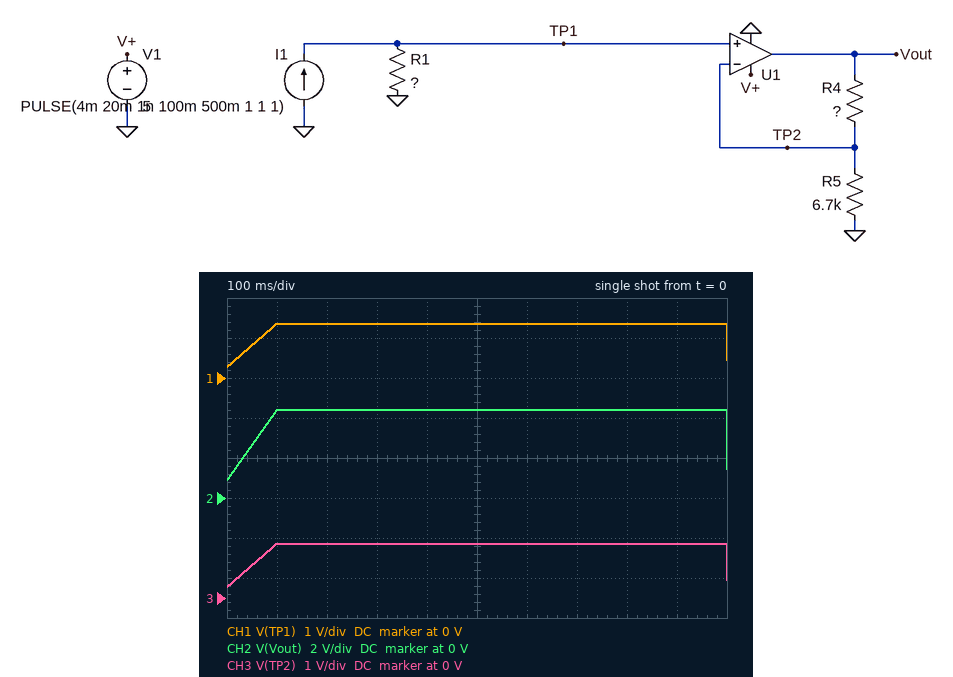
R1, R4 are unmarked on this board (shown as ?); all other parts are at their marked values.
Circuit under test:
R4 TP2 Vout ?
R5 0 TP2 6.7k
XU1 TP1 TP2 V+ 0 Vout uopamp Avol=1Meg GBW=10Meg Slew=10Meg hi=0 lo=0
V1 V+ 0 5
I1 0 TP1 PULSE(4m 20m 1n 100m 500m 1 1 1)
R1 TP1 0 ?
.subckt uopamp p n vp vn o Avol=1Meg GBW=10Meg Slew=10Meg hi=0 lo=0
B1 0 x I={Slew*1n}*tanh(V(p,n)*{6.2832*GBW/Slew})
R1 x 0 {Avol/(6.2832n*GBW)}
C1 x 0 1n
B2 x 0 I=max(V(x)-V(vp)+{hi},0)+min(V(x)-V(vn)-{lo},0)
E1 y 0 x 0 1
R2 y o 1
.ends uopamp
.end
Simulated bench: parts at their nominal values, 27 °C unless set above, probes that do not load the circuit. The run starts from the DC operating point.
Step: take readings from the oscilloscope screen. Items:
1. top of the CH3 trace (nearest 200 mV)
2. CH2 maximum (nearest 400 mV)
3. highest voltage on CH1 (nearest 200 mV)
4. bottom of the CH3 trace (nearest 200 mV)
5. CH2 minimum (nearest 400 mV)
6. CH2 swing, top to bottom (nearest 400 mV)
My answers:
1.4 V
4.4 V
1.4 V
200 mV
800 mV
3.6 V
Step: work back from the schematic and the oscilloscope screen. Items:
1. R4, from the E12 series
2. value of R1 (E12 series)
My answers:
15 kΩ
68 Ω
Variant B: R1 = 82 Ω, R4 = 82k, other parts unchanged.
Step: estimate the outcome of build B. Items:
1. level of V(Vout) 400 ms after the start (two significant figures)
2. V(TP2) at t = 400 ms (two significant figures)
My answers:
5.0 V
380 mV
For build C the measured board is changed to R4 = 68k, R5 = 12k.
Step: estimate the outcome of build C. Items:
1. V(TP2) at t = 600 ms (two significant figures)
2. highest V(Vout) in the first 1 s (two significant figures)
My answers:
750 mV
5.0 V
